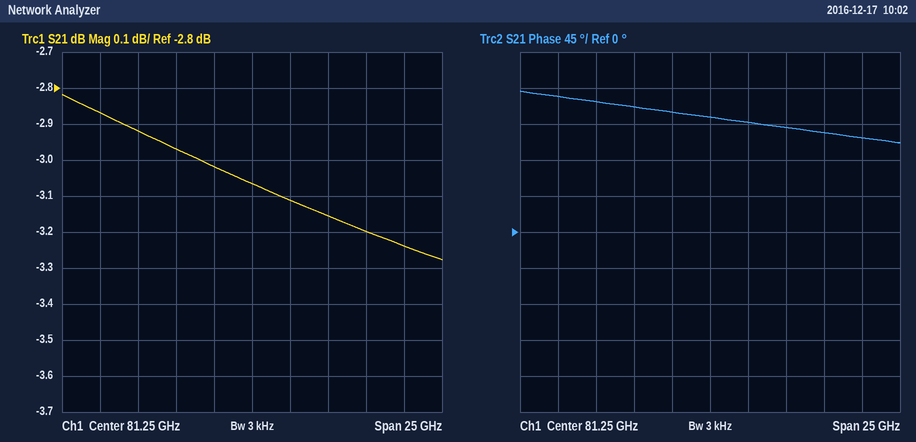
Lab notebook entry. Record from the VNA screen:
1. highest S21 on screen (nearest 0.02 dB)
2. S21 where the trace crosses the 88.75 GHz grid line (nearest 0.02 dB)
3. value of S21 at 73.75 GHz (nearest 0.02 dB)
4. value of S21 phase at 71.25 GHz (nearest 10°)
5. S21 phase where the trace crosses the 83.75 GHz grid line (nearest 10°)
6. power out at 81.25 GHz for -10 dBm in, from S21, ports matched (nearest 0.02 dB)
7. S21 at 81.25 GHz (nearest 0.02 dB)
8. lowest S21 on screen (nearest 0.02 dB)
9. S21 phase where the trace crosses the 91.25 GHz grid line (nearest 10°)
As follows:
-2.82 dB
-3.20 dB
-2.92 dB
170°
140°
-13.06 dBm
-3.06 dB
-3.28 dB
120°
